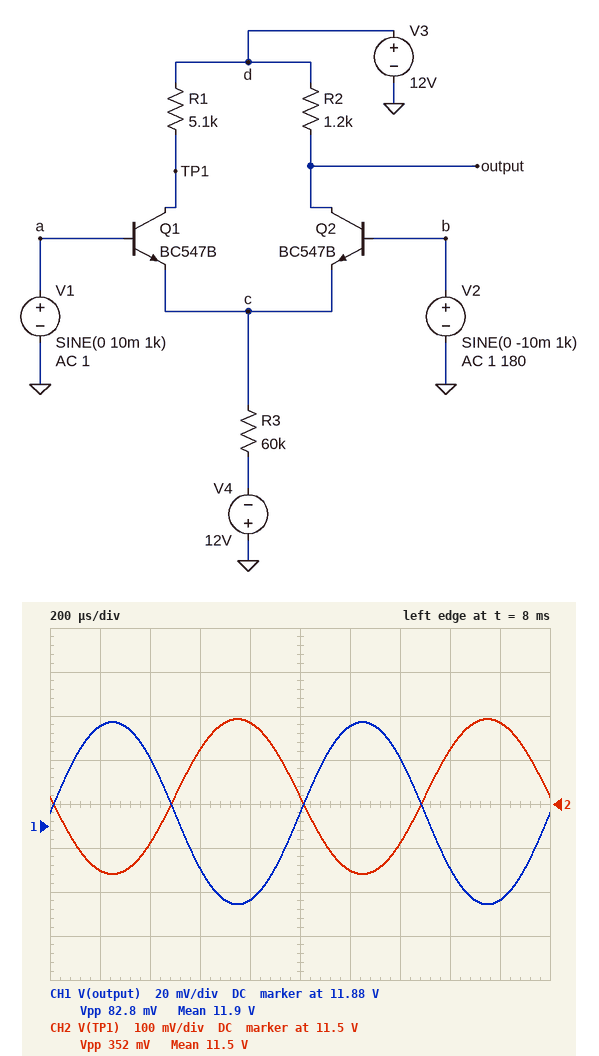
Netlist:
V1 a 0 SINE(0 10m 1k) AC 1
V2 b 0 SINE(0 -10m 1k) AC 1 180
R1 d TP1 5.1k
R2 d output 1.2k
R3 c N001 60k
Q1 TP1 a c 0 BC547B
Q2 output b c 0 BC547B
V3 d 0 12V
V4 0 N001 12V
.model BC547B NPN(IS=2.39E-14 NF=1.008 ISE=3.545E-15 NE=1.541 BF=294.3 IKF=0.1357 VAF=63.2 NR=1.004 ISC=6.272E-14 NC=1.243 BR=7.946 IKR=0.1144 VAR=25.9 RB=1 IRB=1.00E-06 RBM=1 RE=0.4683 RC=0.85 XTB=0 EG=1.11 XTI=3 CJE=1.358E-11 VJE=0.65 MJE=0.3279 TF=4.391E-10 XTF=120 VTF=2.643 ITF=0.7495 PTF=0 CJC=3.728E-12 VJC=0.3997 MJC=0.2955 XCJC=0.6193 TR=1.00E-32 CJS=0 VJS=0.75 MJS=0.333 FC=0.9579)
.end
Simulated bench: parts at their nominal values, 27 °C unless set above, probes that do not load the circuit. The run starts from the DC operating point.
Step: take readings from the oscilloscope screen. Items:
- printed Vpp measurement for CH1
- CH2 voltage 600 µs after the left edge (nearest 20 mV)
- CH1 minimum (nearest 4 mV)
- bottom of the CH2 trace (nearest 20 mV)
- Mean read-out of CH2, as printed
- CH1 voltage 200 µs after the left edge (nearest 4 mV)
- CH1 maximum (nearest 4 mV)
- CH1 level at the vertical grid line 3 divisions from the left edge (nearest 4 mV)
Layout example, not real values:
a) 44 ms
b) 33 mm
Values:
a) 82.8 mV
b) 11.62 V
c) 11.844 V
d) 11.34 V
e) 11.5 V
f) 11.924 V
g) 11.928 V
h) 11.860 V
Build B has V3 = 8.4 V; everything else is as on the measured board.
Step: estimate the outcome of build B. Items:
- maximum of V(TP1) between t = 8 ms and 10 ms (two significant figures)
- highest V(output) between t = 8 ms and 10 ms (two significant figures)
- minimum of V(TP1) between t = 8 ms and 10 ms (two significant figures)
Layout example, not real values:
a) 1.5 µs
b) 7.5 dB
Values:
a) 8.1 V
b) 8.3 V
c) 7.7 V
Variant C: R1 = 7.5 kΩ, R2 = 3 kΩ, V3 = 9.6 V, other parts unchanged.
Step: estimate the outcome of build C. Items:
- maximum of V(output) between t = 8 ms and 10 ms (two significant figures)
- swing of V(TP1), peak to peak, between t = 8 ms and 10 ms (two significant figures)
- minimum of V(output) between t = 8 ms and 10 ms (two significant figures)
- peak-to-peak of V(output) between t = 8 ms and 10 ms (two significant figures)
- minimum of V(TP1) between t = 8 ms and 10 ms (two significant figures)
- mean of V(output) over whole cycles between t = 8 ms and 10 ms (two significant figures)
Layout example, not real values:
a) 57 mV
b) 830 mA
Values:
a) 9.4 V
b) 520 mV
c) 9.2 V
d) 210 mV
e) 8.6 V
f) 9.3 V
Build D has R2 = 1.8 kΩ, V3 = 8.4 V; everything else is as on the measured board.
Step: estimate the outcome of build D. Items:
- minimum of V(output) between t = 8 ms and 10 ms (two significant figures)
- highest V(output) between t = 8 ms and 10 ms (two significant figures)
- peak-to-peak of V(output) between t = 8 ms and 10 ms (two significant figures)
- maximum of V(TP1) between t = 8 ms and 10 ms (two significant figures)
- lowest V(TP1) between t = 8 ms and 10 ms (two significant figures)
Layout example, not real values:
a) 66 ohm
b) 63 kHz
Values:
a) 8.2 V
b) 8.3 V
c) 120 mV
d) 8.1 V
e) 7.7 V
